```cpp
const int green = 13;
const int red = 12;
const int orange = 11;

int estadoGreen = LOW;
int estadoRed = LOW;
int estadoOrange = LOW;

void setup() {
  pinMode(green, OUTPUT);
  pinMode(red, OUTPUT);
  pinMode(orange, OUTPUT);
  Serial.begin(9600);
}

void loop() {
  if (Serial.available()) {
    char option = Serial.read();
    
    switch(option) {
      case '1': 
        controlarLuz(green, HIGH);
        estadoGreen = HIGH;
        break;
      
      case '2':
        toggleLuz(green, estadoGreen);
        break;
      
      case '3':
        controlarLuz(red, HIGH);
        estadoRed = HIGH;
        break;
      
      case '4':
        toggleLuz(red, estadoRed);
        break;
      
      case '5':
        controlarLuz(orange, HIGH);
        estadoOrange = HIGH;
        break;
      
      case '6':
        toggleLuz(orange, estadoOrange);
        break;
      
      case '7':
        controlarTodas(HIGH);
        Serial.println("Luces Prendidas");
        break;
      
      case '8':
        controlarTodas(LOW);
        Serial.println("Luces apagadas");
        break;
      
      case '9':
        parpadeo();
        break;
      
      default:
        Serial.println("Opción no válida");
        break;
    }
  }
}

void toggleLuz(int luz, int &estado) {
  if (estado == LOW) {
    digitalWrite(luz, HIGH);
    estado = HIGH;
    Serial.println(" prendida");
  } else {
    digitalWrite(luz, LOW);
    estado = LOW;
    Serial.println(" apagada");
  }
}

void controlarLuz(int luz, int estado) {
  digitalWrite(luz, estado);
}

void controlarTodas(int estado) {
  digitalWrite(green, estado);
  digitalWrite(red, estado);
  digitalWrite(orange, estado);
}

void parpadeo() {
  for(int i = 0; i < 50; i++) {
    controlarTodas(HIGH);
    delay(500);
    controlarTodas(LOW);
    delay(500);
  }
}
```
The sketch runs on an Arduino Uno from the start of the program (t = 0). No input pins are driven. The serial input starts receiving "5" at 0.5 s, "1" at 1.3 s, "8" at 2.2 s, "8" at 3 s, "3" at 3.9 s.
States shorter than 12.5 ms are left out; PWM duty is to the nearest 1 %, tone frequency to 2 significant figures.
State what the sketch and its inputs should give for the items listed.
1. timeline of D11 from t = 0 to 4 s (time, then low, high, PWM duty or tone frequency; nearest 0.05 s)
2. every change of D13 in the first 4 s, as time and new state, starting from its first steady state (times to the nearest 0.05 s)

0 s low; 0.5 s high; 2.2 s low
0 s low; 1.3 s high; 2.2 s low
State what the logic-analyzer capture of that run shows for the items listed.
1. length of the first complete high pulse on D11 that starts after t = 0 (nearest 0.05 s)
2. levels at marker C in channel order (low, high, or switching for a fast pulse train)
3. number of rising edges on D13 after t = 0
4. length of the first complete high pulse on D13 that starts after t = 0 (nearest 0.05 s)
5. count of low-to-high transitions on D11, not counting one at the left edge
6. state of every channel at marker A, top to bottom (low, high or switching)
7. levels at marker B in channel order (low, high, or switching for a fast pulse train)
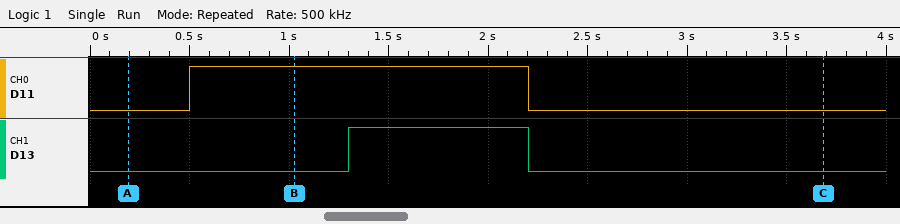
1.70 s
D11 low, D13 low
1
0.90 s
1
D11 low, D13 low
D11 high, D13 low
